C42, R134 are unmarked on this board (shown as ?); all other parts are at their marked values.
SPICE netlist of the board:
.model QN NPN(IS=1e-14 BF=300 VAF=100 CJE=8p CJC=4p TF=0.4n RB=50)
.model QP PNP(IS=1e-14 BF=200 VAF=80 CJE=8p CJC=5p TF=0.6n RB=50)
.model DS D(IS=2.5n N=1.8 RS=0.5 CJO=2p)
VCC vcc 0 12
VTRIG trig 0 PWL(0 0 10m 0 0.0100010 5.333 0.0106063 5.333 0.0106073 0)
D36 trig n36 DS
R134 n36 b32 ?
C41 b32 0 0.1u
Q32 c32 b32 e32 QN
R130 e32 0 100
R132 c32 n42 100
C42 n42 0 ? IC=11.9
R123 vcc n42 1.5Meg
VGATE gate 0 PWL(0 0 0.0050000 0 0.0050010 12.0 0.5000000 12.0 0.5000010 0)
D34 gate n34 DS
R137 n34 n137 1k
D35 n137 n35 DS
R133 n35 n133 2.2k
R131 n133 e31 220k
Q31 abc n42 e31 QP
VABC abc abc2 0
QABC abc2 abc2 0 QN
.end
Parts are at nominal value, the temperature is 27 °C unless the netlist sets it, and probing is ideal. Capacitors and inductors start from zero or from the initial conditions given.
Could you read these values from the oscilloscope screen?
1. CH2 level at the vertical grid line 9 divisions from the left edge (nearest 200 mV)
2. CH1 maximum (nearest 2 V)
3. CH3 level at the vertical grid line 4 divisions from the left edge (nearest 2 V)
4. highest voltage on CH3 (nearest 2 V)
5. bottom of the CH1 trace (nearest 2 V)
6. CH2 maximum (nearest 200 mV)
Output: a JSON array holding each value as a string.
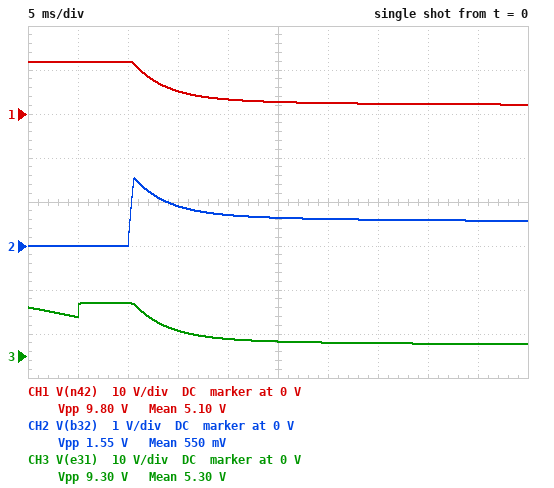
["600 mV", "12 V", "4 V", "12 V", "2 V", "1.6 V"]
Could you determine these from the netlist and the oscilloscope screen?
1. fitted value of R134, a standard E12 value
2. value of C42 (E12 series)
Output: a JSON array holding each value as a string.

["15 kΩ", "3.3 µF"]
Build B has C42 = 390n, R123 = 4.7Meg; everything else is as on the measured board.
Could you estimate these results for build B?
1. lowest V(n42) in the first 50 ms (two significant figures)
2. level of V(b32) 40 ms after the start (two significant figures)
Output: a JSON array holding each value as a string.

["39 mV", "500 mV"]
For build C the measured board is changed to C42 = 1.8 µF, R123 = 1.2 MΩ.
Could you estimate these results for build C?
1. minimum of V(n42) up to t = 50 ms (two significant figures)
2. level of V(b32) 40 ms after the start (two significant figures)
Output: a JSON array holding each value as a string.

["70 mV", "510 mV"]
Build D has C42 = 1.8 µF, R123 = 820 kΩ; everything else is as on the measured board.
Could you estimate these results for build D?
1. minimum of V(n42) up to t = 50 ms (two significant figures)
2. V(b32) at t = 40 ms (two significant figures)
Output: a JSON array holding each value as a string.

["74 mV", "520 mV"]
